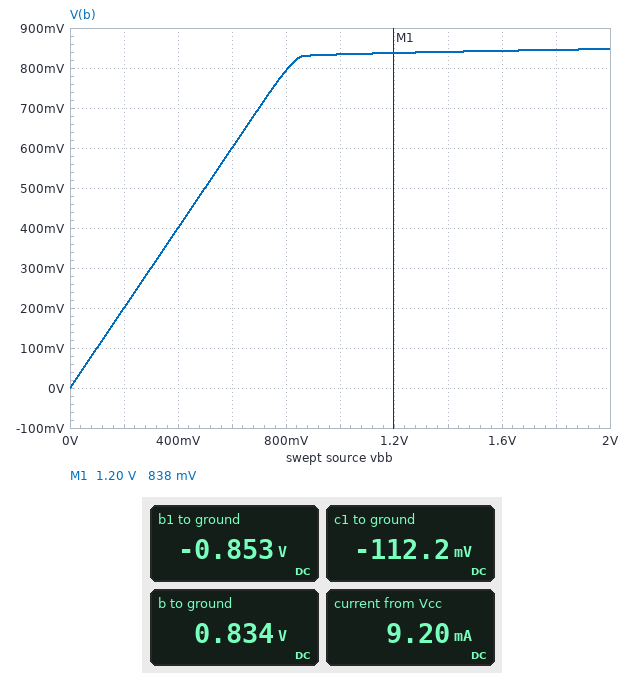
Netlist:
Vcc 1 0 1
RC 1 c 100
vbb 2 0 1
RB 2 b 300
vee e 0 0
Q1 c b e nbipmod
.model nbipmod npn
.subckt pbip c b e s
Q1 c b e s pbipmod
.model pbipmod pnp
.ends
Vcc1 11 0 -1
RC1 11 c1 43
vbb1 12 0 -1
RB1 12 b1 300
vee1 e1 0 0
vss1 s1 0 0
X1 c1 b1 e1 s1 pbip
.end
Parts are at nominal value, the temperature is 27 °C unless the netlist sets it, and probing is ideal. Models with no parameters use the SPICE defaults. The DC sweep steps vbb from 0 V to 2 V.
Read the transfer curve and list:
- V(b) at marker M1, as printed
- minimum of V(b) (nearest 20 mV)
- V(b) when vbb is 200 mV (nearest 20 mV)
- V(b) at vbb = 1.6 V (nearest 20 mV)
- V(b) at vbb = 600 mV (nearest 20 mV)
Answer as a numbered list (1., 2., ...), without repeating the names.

1. 838 mV
2. 0 V
3. 200 mV
4. 840 mV
5. 600 mV
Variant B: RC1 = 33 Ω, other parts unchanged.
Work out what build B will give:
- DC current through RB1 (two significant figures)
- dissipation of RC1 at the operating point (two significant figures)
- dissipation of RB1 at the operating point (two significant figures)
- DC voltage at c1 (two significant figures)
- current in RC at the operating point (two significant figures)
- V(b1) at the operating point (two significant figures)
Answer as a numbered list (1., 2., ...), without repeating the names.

1. 470 µA
2. 23 mW
3. 66 µW
4. -130 mV
5. 9.2 mA
6. -860 mV
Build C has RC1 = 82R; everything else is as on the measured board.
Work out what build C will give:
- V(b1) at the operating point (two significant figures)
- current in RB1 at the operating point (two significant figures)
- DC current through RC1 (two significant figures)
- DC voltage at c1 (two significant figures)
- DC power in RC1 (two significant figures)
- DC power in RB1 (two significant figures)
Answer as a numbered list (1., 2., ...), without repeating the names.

1. -840 mV
2. 540 µA
3. 11 mA
4. -87 mV
5. 10 mW
6. 87 µW
